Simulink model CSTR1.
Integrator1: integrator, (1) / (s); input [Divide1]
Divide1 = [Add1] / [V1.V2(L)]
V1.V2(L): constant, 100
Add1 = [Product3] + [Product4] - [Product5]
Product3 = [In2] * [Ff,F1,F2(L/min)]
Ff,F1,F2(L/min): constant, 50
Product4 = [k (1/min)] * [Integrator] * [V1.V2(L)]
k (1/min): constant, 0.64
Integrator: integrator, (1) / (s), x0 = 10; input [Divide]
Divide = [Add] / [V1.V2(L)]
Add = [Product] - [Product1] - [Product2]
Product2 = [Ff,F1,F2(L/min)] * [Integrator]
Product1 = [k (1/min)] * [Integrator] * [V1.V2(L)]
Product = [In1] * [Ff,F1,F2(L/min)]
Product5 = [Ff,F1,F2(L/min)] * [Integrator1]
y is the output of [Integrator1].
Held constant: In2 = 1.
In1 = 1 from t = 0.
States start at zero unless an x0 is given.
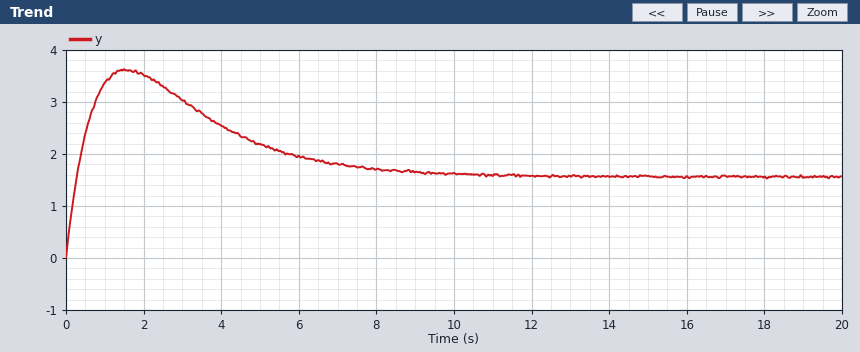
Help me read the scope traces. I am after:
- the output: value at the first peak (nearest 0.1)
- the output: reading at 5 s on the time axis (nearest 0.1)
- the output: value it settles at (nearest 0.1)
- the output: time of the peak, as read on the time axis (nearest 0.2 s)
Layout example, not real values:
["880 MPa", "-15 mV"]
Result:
["3.6", "2.2", "1.6", "1.6 s"]
